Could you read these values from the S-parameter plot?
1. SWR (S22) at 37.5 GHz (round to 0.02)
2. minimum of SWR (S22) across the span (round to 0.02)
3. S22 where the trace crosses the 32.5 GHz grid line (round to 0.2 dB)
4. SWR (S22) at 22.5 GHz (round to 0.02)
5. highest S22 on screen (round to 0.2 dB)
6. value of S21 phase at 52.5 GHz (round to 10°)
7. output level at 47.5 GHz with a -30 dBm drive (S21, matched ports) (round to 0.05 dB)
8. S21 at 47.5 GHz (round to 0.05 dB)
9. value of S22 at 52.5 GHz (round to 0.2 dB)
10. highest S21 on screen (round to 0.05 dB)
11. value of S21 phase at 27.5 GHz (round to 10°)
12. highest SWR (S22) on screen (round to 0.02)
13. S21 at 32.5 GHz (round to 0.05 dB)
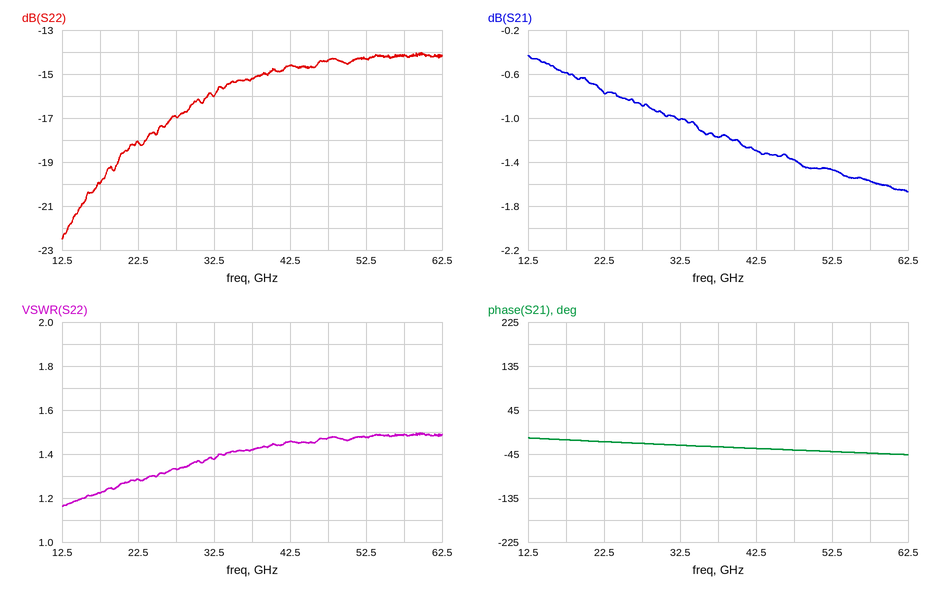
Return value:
1.42
1.16
-16.0 dB
1.28
-14.0 dB
-40°
-31.40 dBm
-1.40 dB
-14.4 dB
-0.45 dB
-20°
1.50
-1.00 dB
